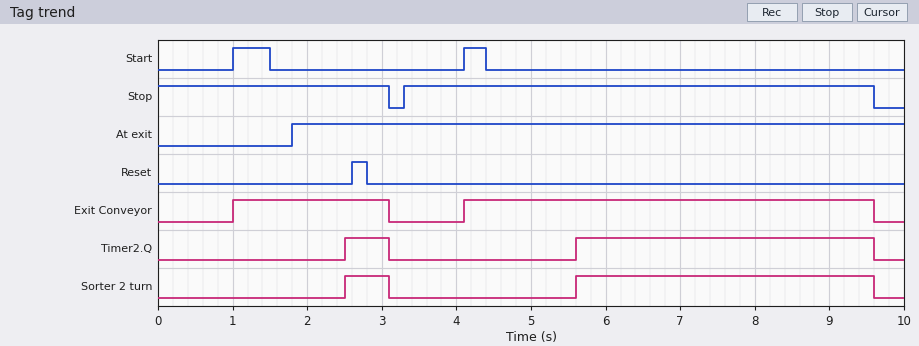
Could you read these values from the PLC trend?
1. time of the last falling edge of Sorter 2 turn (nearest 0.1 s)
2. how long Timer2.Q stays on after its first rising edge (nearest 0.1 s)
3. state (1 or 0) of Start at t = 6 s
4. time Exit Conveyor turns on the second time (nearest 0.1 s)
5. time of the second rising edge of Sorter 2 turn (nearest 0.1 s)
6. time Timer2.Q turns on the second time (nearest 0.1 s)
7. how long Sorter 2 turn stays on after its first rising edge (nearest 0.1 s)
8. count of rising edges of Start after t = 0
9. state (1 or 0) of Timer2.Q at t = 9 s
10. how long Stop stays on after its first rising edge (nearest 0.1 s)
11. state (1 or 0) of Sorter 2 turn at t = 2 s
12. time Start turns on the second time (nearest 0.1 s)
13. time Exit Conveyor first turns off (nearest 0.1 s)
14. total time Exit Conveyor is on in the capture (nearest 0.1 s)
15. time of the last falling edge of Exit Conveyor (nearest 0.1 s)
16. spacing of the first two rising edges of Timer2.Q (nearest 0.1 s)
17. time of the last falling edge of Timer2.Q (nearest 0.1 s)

9.6 s
0.6 s
0
4.1 s
5.6 s
5.6 s
0.6 s
2
1
6.3 s
0
4.1 s
3.1 s
7.6 s
9.6 s
3.1 s
9.6 s
